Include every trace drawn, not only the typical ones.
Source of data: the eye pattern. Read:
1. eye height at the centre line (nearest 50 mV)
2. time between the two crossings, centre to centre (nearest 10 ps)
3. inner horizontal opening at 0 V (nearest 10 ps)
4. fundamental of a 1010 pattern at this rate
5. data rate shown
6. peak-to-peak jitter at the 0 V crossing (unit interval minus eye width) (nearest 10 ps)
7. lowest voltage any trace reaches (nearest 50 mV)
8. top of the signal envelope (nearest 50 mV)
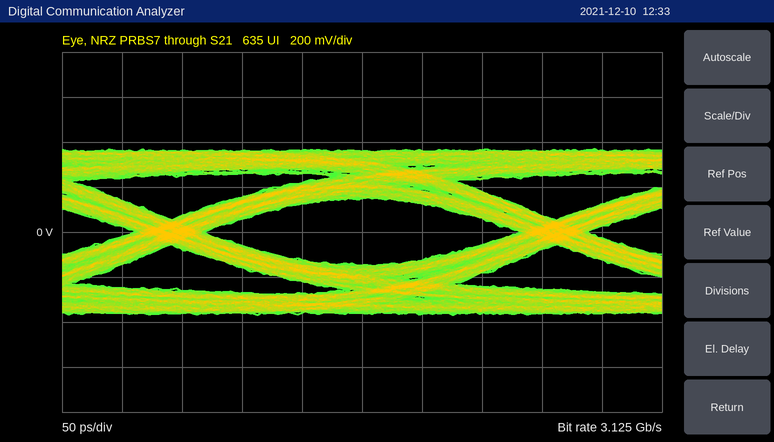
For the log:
300 mV
320 ps
260 ps
1.5625 GHz
3.125 Gb/s
60 ps
-350 mV
350 mV
